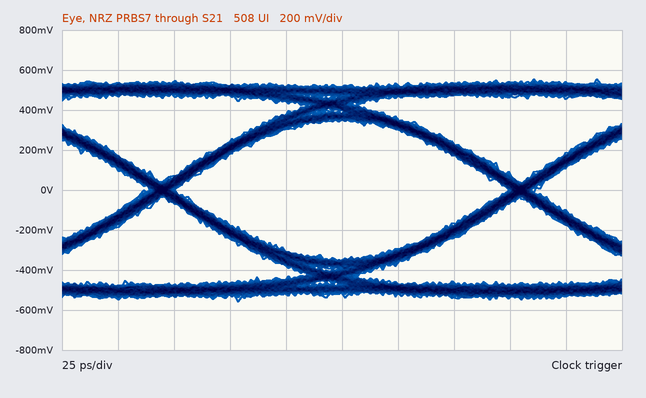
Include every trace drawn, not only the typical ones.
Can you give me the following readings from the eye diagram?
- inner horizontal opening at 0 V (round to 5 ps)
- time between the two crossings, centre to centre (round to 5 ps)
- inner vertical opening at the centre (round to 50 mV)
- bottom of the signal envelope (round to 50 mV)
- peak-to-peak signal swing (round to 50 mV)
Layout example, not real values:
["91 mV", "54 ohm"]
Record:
["150 ps", "160 ps", "700 mV", "-550 mV", "1.10 V"]
